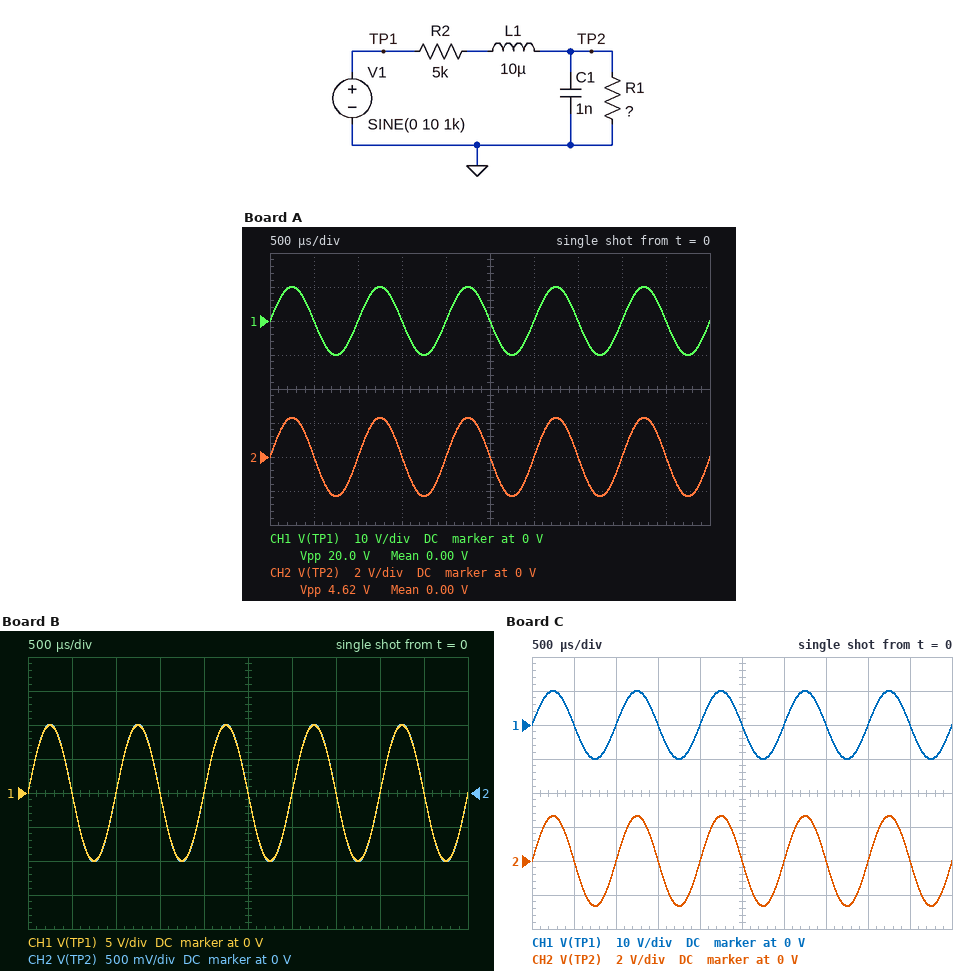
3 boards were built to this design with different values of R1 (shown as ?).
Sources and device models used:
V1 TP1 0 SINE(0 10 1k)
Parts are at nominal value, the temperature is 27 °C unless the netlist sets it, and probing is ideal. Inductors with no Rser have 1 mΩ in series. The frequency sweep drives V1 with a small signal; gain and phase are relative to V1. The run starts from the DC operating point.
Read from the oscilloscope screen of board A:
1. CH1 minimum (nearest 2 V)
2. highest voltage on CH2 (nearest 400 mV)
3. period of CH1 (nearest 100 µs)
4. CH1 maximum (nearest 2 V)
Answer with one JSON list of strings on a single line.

["-10 V", "2.4 V", "1.0 ms", "10 V"]
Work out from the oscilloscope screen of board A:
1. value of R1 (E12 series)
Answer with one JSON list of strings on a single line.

["1.5 kΩ"]
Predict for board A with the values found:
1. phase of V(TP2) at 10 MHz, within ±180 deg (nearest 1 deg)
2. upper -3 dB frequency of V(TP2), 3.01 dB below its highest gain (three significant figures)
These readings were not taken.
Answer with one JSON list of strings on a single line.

["-96 deg", "138 kHz"]
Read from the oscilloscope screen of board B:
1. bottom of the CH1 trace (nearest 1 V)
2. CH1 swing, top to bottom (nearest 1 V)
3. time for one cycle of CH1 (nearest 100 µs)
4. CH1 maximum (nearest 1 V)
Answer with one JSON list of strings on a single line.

["-10 V", "20 V", "1.0 ms", "10 V"]
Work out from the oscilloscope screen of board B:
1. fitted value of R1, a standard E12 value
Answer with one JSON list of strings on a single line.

["560 Ω"]
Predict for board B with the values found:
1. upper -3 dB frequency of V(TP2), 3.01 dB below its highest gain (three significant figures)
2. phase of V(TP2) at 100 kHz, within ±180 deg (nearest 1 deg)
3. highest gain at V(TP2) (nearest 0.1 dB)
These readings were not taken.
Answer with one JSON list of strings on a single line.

["316 kHz", "-18 deg", "-19.9 dB"]
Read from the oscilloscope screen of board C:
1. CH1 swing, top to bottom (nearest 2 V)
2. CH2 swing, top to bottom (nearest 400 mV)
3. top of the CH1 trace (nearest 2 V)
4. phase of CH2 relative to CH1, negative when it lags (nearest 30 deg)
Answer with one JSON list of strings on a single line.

["20 V", "5.2 V", "10 V", "0 deg"]
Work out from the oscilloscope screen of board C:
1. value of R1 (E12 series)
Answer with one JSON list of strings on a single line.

["1.8 kΩ"]
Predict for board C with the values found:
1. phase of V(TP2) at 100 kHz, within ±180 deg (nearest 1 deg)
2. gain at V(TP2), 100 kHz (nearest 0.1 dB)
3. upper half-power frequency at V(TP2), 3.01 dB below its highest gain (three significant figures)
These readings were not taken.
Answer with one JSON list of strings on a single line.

["-40 deg", "-13.8 dB", "120 kHz"]
